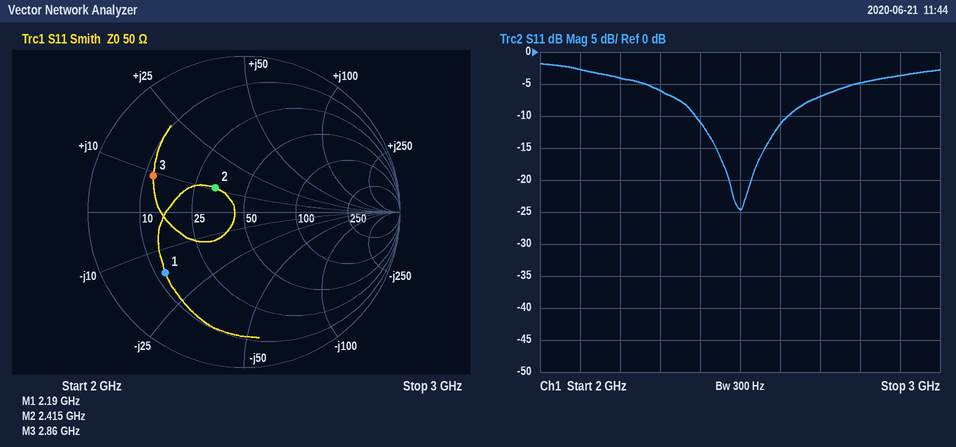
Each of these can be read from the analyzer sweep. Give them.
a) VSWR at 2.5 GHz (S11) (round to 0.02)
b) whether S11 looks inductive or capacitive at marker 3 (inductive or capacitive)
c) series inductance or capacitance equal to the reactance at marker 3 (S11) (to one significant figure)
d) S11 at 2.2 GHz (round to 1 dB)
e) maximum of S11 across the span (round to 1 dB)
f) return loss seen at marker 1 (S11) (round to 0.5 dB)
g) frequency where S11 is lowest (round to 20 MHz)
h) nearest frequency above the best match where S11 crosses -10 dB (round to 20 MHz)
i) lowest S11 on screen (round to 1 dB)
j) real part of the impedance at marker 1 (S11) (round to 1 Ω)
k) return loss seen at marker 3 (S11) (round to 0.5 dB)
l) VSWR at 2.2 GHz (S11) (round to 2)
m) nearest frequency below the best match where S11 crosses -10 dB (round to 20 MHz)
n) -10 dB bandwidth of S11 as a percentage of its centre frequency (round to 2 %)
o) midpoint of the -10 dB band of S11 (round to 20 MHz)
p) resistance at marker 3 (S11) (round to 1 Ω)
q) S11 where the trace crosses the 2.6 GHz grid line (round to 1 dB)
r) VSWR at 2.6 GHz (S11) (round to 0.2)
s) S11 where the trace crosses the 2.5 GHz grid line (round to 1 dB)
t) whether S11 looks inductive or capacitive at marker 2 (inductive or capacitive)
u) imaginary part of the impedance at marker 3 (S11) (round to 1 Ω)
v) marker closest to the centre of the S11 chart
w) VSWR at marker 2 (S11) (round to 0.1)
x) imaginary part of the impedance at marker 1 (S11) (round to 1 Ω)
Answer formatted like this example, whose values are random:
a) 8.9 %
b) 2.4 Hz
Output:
a) 1.12
b) inductive
c) 500 pH
d) -4 dB
e) -2 dB
f) 4.0 dB
g) 2.50 GHz
h) 2.62 GHz
i) -25 dB
j) 12 Ω
k) 4.0 dB
l) 4
m) 2.38 GHz
n) 10 %
o) 2.50 GHz
p) 12 Ω
q) -11 dB
r) 1.8
s) -25 dB
t) inductive
u) +9 Ω
v) marker 2
w) 1.6
x) -16 Ω
